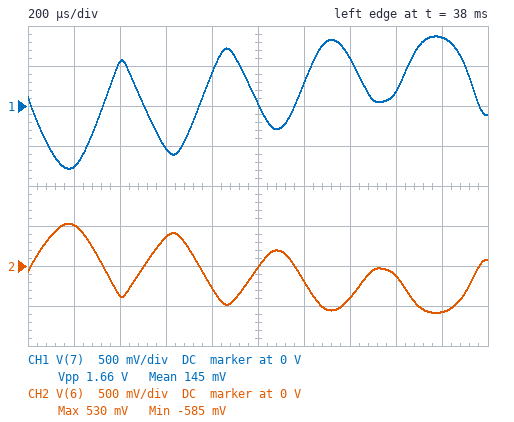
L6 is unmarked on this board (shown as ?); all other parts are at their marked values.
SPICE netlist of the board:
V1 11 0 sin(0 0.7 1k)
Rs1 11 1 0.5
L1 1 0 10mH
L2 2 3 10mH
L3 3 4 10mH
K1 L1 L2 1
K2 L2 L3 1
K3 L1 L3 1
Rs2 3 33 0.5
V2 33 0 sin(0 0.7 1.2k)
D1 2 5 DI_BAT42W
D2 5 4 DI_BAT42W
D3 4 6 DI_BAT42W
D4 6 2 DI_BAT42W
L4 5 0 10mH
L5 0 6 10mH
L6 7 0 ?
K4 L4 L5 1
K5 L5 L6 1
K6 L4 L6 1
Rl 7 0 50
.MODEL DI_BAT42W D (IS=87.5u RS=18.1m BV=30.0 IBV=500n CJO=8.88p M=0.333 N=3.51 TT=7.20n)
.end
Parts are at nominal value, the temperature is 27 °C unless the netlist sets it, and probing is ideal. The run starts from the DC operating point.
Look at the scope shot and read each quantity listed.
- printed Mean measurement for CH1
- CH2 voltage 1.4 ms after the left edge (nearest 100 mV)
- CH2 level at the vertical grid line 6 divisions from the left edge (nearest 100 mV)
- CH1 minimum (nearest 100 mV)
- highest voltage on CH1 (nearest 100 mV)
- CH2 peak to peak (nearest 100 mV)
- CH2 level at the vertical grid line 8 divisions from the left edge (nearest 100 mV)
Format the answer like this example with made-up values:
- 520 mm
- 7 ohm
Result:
- 145 mV
- -400 mV
- -200 mV
- -800 mV
- 900 mV
- 1.1 V
- -100 mV
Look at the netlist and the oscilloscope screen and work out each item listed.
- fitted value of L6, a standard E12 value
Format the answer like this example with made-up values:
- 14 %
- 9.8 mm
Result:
- 22 mH
